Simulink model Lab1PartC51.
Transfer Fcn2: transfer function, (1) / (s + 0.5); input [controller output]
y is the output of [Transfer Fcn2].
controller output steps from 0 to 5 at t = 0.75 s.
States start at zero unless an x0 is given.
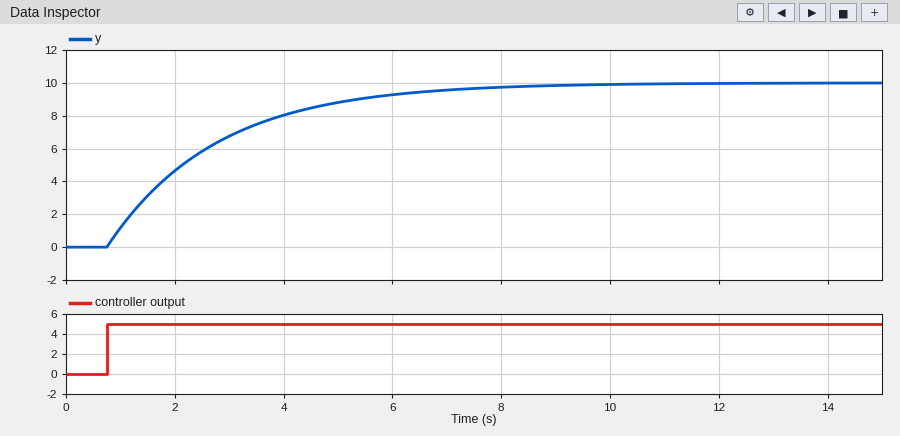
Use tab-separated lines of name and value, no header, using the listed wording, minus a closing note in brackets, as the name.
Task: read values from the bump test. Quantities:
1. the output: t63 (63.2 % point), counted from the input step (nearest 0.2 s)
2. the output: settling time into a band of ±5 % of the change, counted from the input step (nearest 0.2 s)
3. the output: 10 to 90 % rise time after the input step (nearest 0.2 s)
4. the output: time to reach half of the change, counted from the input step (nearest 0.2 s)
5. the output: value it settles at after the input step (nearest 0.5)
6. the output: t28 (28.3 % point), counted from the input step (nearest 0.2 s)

the output: t63 (63.2 % point), counted from the input step	2.0 s
the output: settling time into a band of ±5 % of the change, counted from the input step	6.0 s
the output: 10 to 90 % rise time after the input step	4.4 s
the output: time to reach half of the change, counted from the input step	1.4 s
the output: value it settles at after the input step	10.0
the output: t28 (28.3 % point), counted from the input step	0.6 s
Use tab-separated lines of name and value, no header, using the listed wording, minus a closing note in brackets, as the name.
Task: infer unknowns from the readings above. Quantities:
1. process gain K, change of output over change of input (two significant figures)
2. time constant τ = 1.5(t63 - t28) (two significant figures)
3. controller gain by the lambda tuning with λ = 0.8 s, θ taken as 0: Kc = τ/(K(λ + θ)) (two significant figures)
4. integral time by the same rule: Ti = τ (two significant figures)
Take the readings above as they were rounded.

process gain K, change of output over change of input	2.0
time constant τ = 1.5(t63 - t28)	2.1 s
controller gain by the lambda tuning with λ = 0.8 s, θ taken as 0: Kc = τ/(K(λ + θ))	1.3
integral time by the same rule: Ti = τ	2.1 s
